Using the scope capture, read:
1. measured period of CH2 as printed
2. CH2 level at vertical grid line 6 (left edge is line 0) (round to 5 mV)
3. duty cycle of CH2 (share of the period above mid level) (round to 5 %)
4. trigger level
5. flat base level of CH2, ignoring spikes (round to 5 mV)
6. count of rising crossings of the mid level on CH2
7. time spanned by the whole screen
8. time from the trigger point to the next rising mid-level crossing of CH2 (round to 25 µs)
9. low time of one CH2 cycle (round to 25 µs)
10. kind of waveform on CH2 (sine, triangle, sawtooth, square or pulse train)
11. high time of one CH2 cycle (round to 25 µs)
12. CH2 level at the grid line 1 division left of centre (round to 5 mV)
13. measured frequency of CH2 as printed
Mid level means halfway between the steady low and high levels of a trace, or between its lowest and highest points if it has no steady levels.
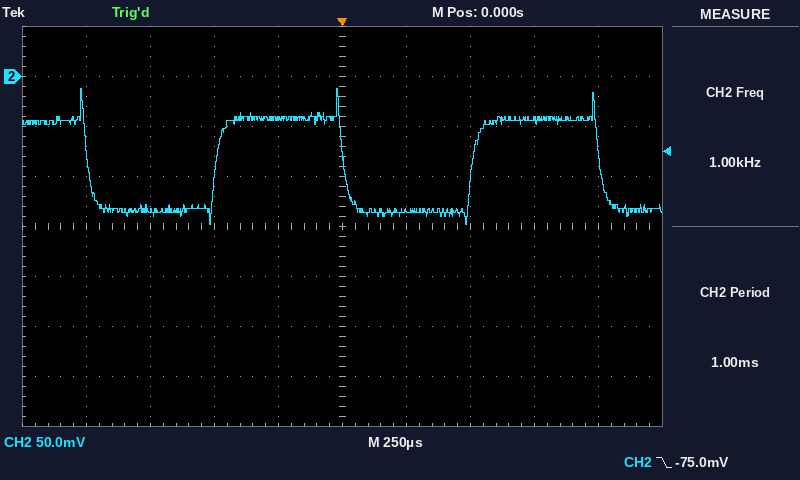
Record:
1.00 ms
-135 mV
50 %
-75.0 mV
-135 mV
2
2.5 ms
500 µs
500 µs
square
500 µs
-40 mV
1.00 kHz
